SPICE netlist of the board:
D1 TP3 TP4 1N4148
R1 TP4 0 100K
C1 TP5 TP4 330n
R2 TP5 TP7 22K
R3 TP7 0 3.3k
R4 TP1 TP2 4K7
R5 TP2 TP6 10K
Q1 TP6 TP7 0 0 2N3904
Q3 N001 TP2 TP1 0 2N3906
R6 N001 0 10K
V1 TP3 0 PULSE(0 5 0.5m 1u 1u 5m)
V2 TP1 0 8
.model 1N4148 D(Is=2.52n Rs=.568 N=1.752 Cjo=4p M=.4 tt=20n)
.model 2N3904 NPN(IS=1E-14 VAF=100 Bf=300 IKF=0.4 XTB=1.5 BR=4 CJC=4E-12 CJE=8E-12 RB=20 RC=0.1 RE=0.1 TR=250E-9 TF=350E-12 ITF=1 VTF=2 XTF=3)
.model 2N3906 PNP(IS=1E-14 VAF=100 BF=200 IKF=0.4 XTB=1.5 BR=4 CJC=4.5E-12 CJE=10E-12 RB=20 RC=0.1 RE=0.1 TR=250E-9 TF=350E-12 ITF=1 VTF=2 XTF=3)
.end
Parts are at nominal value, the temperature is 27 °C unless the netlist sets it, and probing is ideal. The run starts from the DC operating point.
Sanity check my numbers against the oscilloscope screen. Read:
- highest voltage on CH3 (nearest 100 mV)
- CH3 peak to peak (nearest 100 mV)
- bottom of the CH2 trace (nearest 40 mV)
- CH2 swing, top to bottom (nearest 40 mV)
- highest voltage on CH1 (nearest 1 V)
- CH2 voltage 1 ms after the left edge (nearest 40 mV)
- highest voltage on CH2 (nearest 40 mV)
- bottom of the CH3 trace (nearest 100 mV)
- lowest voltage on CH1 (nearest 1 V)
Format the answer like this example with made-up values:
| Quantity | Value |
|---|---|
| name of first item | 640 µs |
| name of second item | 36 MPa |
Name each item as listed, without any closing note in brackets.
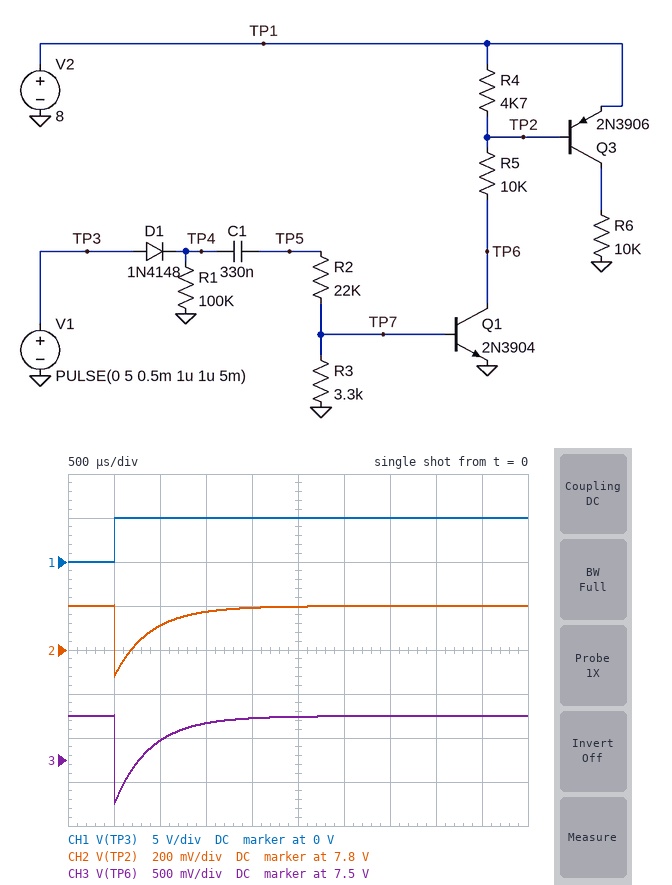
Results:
| Quantity | Value |
|---|---|
| highest voltage on CH3 | 8.0 V |
| CH3 peak to peak | 1.0 V |
| bottom of the CH2 trace | 7.68 V |
| CH2 swing, top to bottom | 320 mV |
| highest voltage on CH1 | 5 V |
| CH2 voltage 1 ms after the left edge | 7.92 V |
| highest voltage on CH2 | 8.00 V |
| bottom of the CH3 trace | 7.0 V |
| lowest voltage on CH1 | 0 V |
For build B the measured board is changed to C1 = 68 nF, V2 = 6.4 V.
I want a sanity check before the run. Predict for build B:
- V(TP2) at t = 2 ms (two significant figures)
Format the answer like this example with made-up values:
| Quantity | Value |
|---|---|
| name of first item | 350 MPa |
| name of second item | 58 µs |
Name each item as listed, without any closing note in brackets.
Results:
| Quantity | Value |
|---|---|
| V(TP2) at t = 2 ms | 6.4 V |
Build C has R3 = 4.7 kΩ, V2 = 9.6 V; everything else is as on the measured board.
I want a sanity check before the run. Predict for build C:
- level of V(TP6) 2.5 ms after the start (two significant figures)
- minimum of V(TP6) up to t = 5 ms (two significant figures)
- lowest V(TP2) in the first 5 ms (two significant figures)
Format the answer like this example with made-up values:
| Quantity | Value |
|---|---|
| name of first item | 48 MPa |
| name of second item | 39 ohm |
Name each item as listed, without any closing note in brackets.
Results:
| Quantity | Value |
|---|---|
| level of V(TP6) 2.5 ms after the start | 5.7 V |
| minimum of V(TP6) up to t = 5 ms | 56 mV |
| lowest V(TP2) in the first 5 ms | 8.9 V |
